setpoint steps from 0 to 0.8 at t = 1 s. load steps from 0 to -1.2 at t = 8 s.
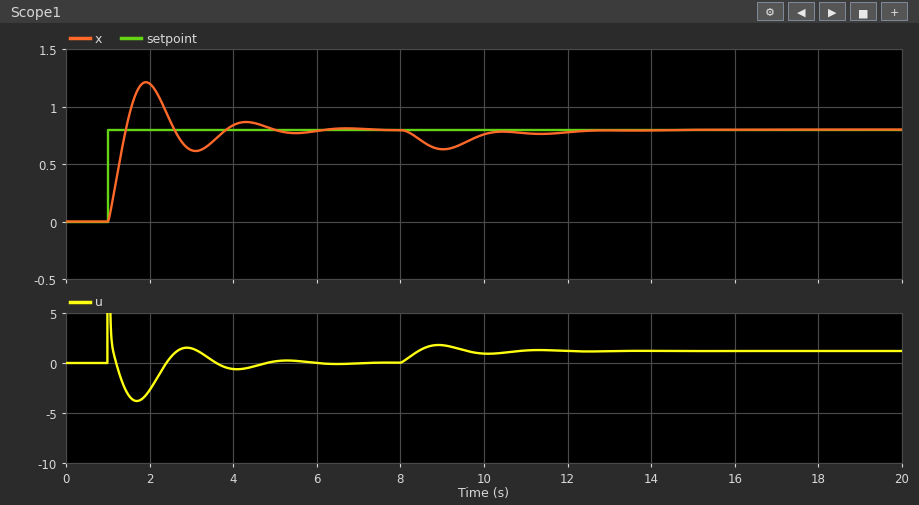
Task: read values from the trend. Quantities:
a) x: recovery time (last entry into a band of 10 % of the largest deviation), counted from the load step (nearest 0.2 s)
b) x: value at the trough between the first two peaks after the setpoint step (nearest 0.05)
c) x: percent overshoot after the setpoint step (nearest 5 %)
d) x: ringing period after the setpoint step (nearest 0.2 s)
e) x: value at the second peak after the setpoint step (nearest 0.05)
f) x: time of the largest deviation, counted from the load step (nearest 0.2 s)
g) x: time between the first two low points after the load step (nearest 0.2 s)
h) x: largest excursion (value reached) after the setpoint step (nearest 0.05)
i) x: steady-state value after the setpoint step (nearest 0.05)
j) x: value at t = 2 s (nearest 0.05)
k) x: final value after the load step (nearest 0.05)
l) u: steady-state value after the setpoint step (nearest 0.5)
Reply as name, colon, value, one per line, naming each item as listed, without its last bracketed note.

x: recovery time (last entry into a band of 10 % of the largest deviation), counted from the load step: 4.2 s
x: value at the trough between the first two peaks after the setpoint step: 0.60
x: percent overshoot after the setpoint step: 50 %
x: ringing period after the setpoint step: 2.4 s
x: value at the second peak after the setpoint step: 0.85
x: time of the largest deviation, counted from the load step: 1.0 s
x: time between the first two low points after the load step: 2.4 s
x: largest excursion (value reached) after the setpoint step: 1.20
x: steady-state value after the setpoint step: 0.80
x: value at t = 2 s: 1.20
x: final value after the load step: 0.80
u: steady-state value after the setpoint step: 0.0
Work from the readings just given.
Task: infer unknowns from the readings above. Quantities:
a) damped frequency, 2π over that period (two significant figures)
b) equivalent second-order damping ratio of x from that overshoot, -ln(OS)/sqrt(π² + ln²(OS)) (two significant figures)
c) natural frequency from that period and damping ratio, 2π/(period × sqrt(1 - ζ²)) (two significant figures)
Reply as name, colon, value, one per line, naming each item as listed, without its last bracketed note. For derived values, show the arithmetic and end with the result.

damped frequency, 2π over that period: 2π / 2.4 = 2.6 rad/s
equivalent second-order damping ratio of x from that overshoot, -ln(OS)/sqrt(π² + ln²(OS)): ln(0.5) = -0.693; 0.693 / sqrt(9.870 + 0.480) = 0.22
natural frequency from that period and damping ratio, 2π/(period × sqrt(1 - ζ²)): 2π / (2.4 × sqrt(1 - 0.22²)) = 2.7 rad/s
